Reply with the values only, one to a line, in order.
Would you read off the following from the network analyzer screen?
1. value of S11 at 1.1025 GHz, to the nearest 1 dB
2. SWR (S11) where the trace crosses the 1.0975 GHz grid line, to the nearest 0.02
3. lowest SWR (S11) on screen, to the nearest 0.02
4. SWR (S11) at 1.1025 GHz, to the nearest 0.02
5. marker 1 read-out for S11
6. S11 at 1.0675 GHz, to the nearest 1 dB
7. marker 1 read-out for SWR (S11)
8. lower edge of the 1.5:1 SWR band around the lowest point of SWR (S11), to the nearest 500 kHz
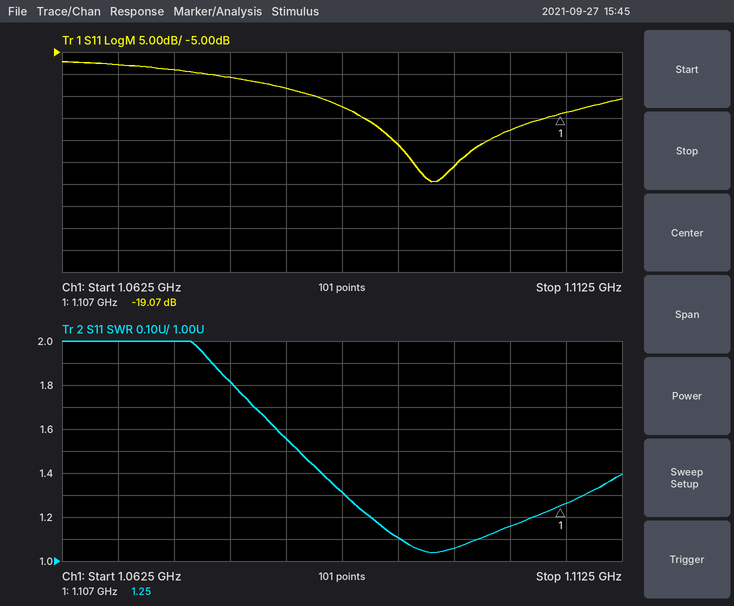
-23 dB
1.06
1.04
1.16
-19.07 dB
-8 dB
1.25
1.0835 GHz
